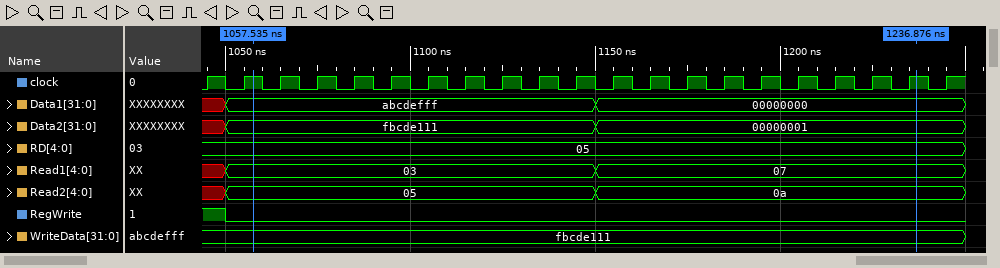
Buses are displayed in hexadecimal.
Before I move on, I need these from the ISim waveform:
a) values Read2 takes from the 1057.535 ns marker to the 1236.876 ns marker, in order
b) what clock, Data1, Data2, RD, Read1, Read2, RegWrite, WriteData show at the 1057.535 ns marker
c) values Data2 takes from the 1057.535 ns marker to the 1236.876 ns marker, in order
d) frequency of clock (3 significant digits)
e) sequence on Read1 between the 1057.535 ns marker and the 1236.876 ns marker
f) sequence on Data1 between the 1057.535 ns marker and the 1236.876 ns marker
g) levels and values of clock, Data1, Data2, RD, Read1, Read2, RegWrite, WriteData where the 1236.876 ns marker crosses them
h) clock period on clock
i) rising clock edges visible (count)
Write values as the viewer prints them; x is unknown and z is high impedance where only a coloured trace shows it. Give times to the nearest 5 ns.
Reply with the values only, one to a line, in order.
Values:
05, 0a
clock=1, Data1=abcdefff, Data2=fbcde111, RD=05, Read1=03, Read2=05, RegWrite=0, WriteData=fbcde111
fbcde111, 00000001
100 MHz
03, 07
abcdefff, 00000000
clock=1, Data1=00000000, Data2=00000001, RD=05, Read1=07, Read2=0a, RegWrite=0, WriteData=fbcde111
10 ns
21
